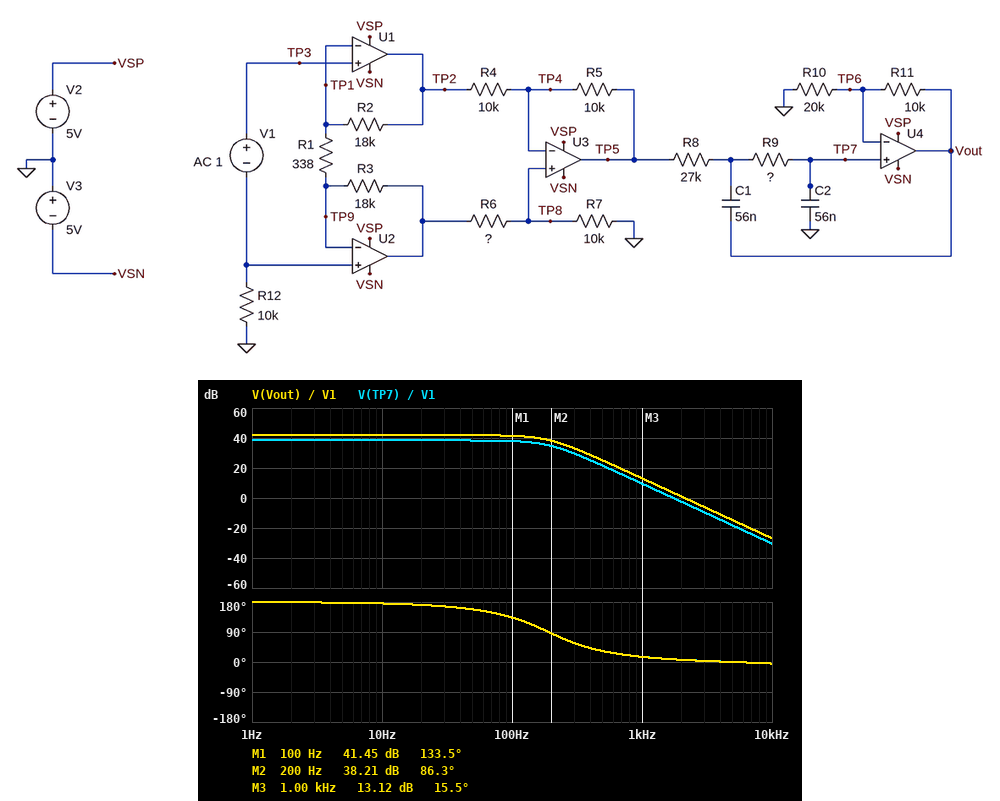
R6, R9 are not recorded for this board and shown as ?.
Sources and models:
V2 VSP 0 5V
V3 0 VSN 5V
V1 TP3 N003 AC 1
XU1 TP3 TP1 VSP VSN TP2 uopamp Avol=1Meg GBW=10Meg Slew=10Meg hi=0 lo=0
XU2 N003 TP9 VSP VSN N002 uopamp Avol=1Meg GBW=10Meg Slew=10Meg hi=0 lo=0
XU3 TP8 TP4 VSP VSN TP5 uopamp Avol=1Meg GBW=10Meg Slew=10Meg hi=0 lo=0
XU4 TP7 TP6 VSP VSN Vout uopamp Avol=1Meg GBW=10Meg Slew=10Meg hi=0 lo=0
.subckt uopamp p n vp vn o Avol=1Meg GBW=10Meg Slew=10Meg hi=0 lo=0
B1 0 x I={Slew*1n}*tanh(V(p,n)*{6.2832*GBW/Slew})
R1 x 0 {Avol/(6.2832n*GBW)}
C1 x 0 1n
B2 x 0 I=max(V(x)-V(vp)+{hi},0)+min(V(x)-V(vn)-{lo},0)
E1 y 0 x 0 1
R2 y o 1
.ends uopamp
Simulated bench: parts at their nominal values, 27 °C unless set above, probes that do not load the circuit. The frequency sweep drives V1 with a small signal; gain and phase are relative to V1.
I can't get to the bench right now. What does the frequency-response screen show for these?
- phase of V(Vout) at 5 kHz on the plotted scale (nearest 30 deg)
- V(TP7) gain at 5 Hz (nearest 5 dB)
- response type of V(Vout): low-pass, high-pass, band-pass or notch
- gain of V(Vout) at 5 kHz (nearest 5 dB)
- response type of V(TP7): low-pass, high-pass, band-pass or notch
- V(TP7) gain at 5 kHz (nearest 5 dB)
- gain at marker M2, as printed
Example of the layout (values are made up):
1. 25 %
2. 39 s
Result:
1. 0 deg
2. 40 dB
3. low-pass
4. -15 dB
5. low-pass
6. -20 dB
7. 38.21 dB
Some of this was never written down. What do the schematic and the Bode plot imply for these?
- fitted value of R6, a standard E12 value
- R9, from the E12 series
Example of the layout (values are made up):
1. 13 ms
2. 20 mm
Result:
1. 27 kΩ
2. 8.2 kΩ
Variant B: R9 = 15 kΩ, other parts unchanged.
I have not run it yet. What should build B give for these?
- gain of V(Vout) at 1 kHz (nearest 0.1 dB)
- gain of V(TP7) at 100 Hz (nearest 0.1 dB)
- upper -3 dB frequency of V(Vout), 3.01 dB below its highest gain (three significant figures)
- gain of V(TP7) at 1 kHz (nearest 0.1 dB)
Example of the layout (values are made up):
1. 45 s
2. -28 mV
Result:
1. 7.9 dB
2. 37.4 dB
3. 141 Hz
4. 4.4 dB
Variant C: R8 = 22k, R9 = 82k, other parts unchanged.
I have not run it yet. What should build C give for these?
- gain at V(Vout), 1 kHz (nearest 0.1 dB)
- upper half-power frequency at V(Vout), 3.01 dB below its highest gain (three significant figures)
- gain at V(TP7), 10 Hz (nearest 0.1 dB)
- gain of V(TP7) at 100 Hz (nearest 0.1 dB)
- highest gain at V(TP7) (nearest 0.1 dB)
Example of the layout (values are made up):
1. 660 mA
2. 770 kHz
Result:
1. -5.1 dB
2. 37.9 Hz
3. 38.1 dB
4. 27.5 dB
5. 38.4 dB
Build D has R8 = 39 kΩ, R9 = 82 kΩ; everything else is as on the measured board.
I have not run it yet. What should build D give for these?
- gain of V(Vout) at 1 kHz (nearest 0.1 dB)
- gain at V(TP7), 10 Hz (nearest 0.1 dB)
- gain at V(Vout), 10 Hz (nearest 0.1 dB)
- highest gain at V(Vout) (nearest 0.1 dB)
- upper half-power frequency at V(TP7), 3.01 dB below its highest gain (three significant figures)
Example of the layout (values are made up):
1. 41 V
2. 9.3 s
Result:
1. -10.1 dB
2. 38.2 dB
3. 41.7 dB
4. 41.9 dB
5. 37.6 Hz
